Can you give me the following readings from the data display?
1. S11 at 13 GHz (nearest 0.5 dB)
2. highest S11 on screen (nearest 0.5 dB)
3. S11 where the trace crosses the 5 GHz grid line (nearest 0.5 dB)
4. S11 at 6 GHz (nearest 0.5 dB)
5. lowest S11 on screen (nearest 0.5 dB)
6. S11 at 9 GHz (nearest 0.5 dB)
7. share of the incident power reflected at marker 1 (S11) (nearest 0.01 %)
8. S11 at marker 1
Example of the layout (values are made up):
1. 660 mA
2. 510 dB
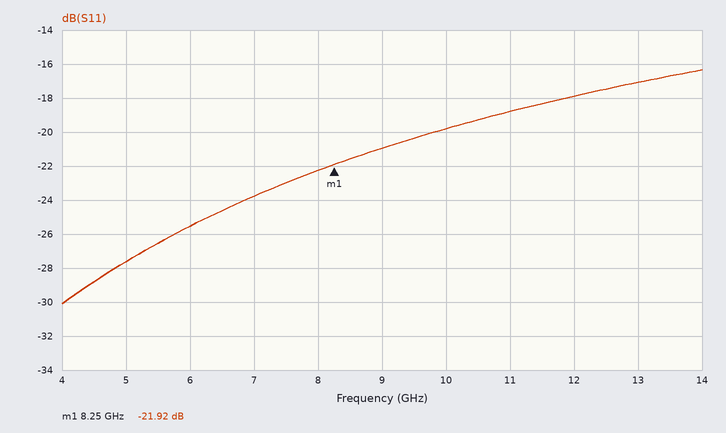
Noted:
1. -17.0 dB
2. -16.5 dB
3. -27.5 dB
4. -25.5 dB
5. -30.0 dB
6. -21.0 dB
7. 0.64 %
8. -21.92 dB
